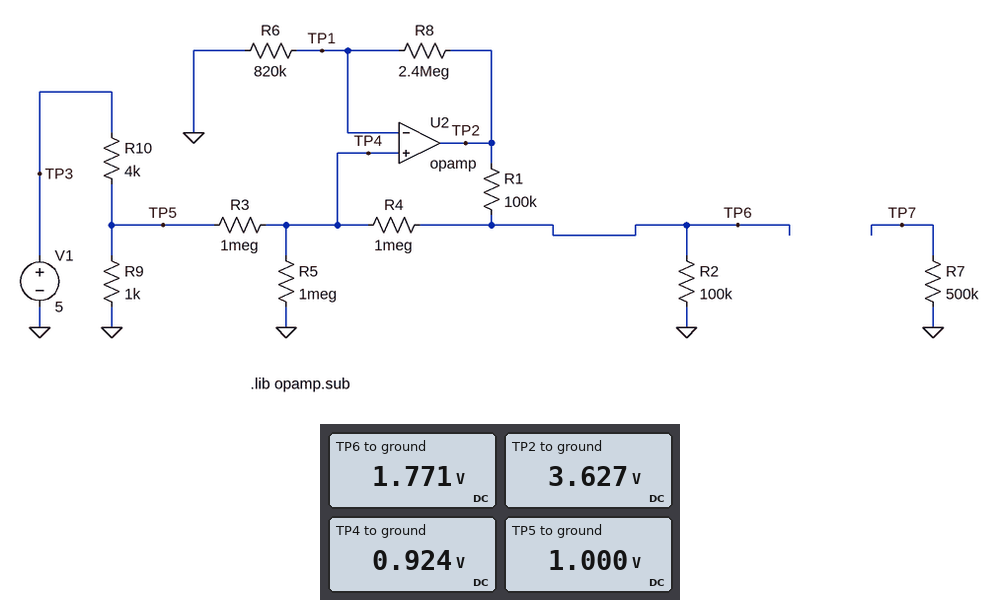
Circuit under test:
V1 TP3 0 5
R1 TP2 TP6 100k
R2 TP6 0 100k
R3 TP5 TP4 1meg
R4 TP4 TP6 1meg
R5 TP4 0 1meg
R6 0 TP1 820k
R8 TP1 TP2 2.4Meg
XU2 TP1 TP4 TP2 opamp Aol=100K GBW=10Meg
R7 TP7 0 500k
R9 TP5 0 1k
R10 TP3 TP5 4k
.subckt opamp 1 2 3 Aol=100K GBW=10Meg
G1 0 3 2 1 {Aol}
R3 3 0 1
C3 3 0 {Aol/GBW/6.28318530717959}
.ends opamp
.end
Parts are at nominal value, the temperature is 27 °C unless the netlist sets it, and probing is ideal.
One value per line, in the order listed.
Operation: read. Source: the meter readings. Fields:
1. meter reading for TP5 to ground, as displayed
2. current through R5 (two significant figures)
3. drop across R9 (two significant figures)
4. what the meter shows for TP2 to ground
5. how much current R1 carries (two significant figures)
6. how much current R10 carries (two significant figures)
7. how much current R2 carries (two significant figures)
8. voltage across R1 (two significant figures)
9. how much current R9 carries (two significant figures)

1.000 V
920 nA
1.0 V
3.627 V
19 µA
1.0 mA
18 µA
1.9 V
1.0 mA
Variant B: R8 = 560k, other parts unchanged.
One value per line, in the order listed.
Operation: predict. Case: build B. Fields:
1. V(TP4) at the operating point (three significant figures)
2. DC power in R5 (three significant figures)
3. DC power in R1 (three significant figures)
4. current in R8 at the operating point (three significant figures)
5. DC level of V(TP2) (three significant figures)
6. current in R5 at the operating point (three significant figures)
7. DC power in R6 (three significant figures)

465 mV
216 nW
1.50 µW
567 nA
782 mV
465 nA
263 nW
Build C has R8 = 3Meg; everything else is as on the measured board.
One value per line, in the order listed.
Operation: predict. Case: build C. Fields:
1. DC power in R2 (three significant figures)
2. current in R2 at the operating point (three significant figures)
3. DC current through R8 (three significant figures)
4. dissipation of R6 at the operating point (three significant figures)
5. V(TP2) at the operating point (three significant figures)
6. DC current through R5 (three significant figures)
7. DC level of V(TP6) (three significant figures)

95.3 µW
30.9 µA
1.66 µA
2.26 µW
6.35 V
1.36 µA
3.09 V
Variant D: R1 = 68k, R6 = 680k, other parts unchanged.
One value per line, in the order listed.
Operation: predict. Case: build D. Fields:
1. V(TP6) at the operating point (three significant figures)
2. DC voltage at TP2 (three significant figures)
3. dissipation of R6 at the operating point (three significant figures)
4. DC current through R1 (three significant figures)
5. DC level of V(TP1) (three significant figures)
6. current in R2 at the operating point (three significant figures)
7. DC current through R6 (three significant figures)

7.12 V
12.3 V
10.8 µW
75.6 µA
2.71 V
71.2 µA
3.98 µA
